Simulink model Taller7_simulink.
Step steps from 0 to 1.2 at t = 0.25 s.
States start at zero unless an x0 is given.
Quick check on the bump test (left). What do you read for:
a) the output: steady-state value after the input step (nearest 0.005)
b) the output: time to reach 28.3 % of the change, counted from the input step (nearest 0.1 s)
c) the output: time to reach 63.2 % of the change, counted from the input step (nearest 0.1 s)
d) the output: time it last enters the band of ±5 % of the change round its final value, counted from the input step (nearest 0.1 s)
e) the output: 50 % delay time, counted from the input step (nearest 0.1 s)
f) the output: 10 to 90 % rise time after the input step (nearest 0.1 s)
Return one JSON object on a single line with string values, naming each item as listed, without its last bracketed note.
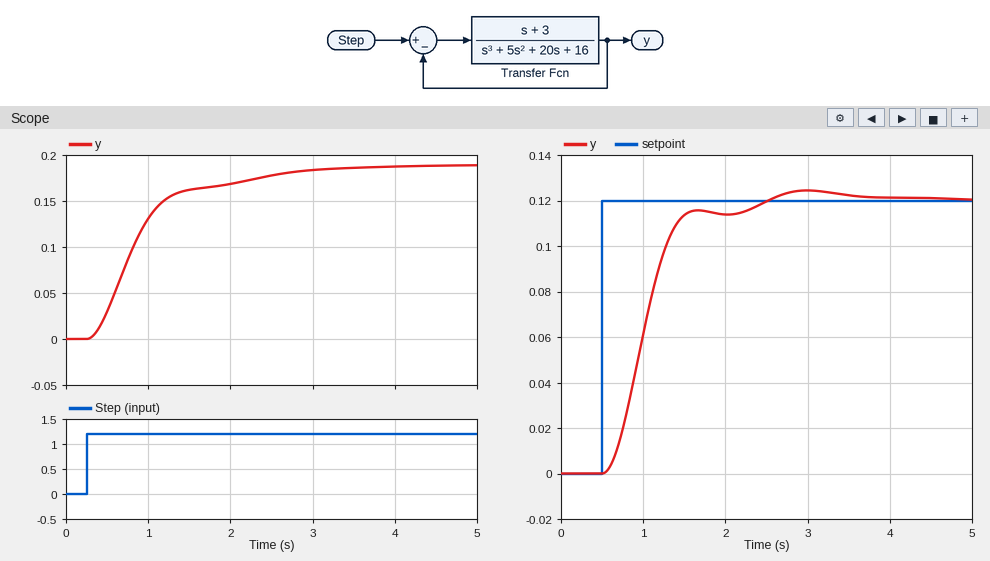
{"the output: steady-state value after the input step": "0.190", "the output: time to reach 28.3 % of the change, counted from the input step": "0.4 s", "the output: time to reach 63.2 % of the change, counted from the input step": "0.7 s", "the output: time it last enters the band of ±5 % of the change round its final value, counted from the input step": "2.4 s", "the output: 50 % delay time, counted from the input step": "0.5 s", "the output: 10 to 90 % rise time after the input step": "1.7 s"}
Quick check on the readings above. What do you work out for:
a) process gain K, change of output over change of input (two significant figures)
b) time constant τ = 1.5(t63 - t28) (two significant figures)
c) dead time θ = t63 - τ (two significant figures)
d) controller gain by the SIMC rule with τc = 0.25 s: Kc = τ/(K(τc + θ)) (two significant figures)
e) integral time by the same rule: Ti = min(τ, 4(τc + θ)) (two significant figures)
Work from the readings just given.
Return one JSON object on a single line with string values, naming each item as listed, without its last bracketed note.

{"process gain K, change of output over change of input": "0.16", "time constant τ = 1.5(t63 - t28)": "0.45 s", "dead time θ = t63 - τ": "0.25 s", "controller gain by the SIMC rule with τc = 0.25 s: Kc = τ/(K(τc + θ))": "5.6", "integral time by the same rule: Ti = min(τ, 4(τc + θ))": "0.45 s"}
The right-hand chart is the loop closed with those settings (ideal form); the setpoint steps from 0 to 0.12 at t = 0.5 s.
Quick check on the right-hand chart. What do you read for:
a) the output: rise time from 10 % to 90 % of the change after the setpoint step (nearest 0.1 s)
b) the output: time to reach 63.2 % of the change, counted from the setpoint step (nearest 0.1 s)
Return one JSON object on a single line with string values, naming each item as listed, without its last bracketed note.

{"the output: rise time from 10 % to 90 % of the change after the setpoint step": "0.7 s", "the output: time to reach 63.2 % of the change, counted from the setpoint step": "0.6 s"}
